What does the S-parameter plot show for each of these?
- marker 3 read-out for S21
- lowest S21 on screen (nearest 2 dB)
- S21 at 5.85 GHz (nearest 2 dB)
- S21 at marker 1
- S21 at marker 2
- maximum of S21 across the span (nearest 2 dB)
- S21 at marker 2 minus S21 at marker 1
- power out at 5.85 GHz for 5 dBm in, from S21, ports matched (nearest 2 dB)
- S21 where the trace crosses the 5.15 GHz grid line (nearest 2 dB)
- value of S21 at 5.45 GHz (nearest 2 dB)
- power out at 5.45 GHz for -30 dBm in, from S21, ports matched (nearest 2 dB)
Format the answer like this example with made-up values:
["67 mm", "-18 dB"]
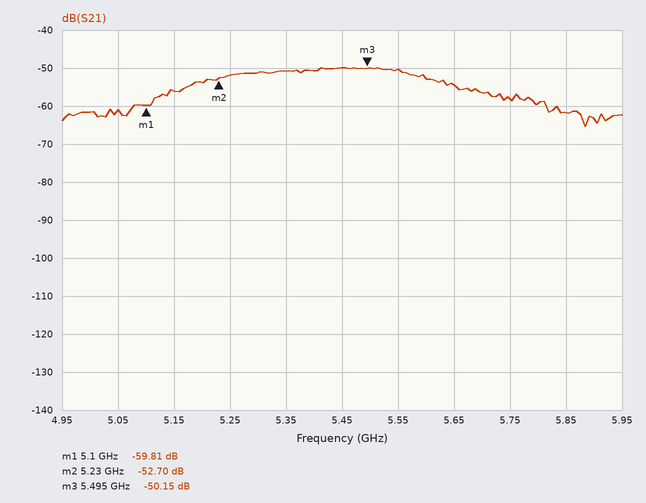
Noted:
["-50.15 dB", "-66 dB", "-62 dB", "-59.81 dB", "-52.70 dB", "-50 dB", "7.11 dB", "-56 dBm", "-56 dB", "-50 dB", "-80 dBm"]
